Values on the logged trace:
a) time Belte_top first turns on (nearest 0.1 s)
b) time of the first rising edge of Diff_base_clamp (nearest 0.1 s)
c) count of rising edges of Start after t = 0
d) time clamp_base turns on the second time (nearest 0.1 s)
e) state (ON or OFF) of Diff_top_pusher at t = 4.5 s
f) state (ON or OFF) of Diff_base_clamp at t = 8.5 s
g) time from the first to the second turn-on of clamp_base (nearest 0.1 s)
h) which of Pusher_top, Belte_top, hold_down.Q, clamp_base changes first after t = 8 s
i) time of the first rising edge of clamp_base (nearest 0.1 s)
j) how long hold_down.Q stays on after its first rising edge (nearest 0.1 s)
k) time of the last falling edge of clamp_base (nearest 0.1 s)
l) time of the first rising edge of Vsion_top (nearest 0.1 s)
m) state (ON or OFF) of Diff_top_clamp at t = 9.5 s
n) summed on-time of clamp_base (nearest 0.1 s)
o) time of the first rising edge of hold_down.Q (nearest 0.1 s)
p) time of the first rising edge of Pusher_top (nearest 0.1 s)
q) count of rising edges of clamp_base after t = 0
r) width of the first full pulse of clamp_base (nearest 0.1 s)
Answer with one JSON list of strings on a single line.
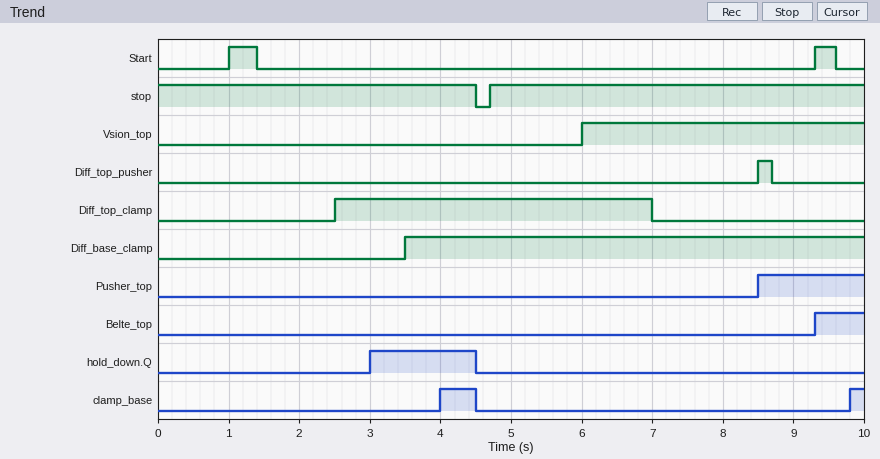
["9.3 s", "3.5 s", "2", "9.8 s", "OFF", "ON", "5.8 s", "Pusher_top", "4.0 s", "1.5 s", "4.5 s", "6.0 s", "OFF", "0.7 s", "3.0 s", "8.5 s", "2", "0.5 s"]
